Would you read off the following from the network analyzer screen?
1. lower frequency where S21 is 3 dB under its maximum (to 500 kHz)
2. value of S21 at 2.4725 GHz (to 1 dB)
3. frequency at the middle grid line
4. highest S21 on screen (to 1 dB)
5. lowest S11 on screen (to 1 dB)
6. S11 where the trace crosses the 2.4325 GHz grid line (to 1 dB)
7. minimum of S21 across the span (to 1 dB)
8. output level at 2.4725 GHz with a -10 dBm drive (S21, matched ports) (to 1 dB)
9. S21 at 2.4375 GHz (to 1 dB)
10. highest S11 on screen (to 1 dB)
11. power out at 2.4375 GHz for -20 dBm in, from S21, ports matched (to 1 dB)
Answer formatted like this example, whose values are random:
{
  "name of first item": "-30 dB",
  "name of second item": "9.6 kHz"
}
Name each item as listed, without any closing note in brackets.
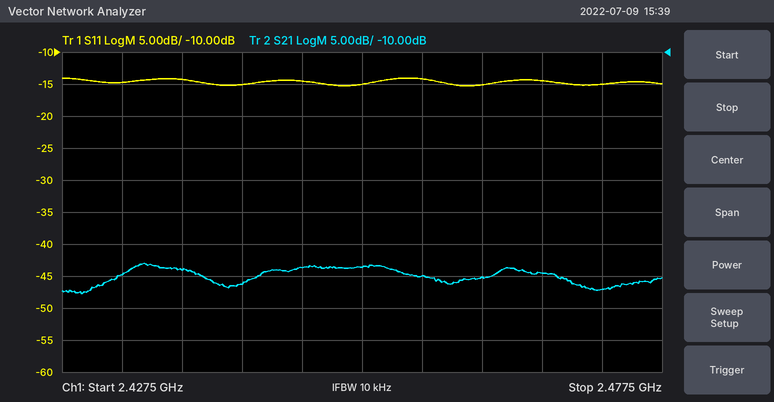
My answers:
{
  "lower frequency where S21 is 3 dB under its maximum": "2.4310 GHz",
  "value of S21 at 2.4725 GHz": "-47 dB",
  "frequency at the middle grid line": "2.4525 GHz",
  "highest S21 on screen": "-43 dB",
  "lowest S11 on screen": "-15 dB",
  "S11 where the trace crosses the 2.4325 GHz grid line": "-15 dB",
  "minimum of S21 across the span": "-48 dB",
  "output level at 2.4725 GHz with a -10 dBm drive (S21, matched ports)": "-57 dBm",
  "S21 at 2.4375 GHz": "-44 dB",
  "highest S11 on screen": "-14 dB",
  "power out at 2.4375 GHz for -20 dBm in, from S21, ports matched": "-64 dBm"
}
